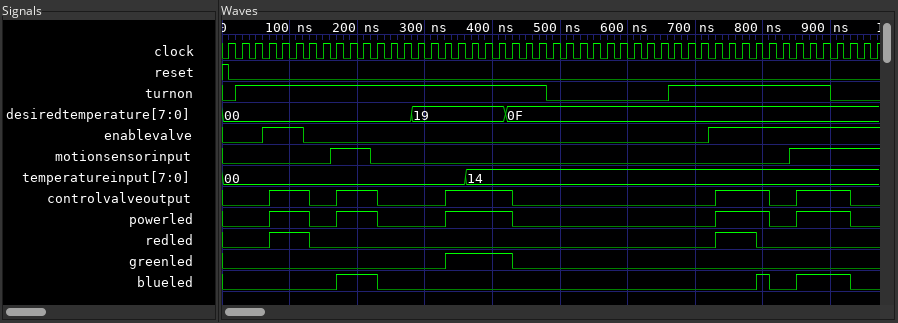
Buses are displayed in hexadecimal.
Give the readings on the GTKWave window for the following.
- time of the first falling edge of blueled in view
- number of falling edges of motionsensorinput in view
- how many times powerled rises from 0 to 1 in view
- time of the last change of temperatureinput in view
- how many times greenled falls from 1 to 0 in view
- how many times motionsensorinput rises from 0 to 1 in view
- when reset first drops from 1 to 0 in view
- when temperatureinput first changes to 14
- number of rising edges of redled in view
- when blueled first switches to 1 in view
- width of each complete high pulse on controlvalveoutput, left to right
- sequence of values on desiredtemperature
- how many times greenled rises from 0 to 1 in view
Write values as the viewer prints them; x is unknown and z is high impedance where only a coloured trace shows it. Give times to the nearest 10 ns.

230 ns
1
5
360 ns
1
2
10 ns
360 ns
2
170 ns
60 ns, 60 ns, 100 ns, 80 ns, 80 ns
00, 19, 0F
1
